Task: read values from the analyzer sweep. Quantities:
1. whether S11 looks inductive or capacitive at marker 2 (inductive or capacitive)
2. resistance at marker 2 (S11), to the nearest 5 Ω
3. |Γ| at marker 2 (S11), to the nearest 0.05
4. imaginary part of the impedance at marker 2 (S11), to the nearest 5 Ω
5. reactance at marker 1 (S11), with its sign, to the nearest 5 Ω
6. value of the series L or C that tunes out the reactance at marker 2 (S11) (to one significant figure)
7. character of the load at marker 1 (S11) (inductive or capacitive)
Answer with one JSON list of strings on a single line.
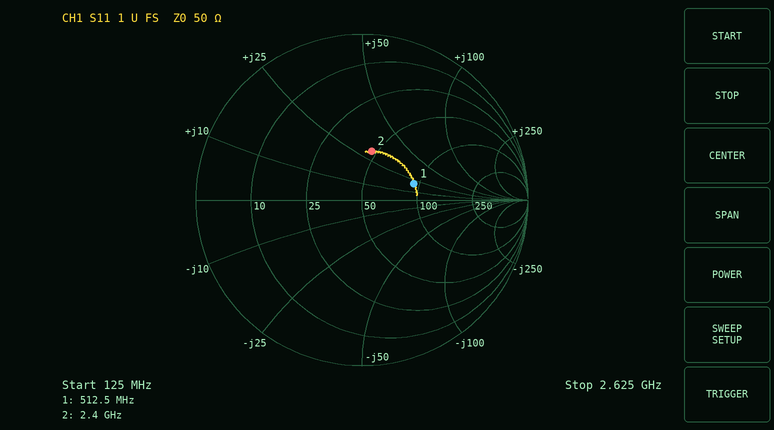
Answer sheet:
["inductive", "45 Ω", "0.30", "+30 Ω", "+20 Ω", "2 pF", "inductive"]
